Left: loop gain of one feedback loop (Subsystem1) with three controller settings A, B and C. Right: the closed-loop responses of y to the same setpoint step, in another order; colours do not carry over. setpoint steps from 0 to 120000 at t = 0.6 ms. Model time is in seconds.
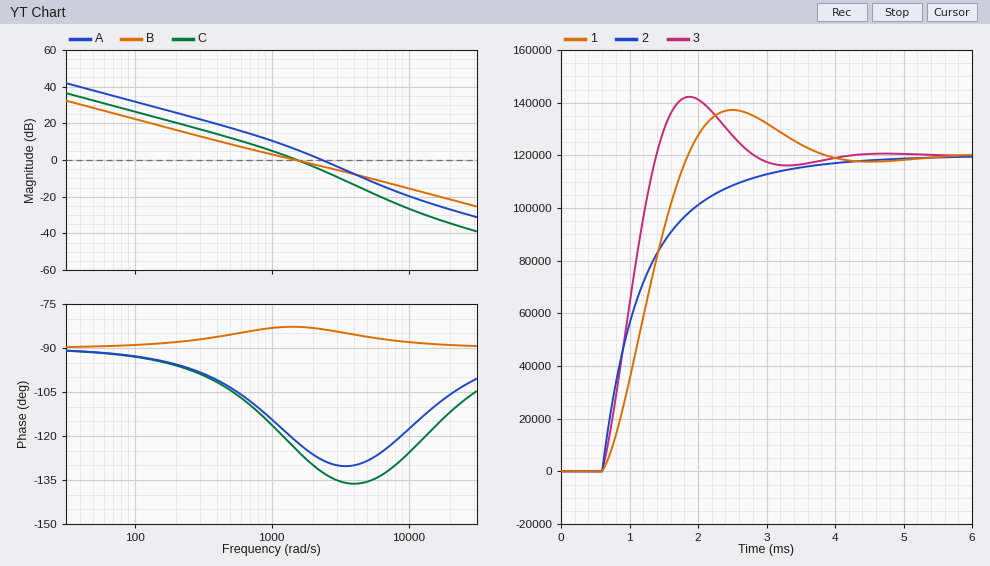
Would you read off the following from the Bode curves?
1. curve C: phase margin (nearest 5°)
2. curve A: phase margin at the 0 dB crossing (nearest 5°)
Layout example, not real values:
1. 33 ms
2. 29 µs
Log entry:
1. 55°
2. 50°
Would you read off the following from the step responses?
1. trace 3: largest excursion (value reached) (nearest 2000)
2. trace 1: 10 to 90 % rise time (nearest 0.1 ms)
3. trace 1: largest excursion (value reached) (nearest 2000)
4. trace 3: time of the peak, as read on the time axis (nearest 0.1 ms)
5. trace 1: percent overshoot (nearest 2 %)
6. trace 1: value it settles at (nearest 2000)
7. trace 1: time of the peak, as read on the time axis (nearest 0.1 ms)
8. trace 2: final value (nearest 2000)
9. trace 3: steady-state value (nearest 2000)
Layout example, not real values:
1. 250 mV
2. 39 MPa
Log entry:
1. 142000
2. 0.9 ms
3. 138000
4. 1.9 ms
5. 14 %
6. 120000
7. 2.5 ms
8. 120000
9. 120000
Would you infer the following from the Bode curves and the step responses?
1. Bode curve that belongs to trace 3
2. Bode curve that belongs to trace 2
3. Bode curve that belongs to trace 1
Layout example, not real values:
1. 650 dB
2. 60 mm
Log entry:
1. A
2. B
3. C
